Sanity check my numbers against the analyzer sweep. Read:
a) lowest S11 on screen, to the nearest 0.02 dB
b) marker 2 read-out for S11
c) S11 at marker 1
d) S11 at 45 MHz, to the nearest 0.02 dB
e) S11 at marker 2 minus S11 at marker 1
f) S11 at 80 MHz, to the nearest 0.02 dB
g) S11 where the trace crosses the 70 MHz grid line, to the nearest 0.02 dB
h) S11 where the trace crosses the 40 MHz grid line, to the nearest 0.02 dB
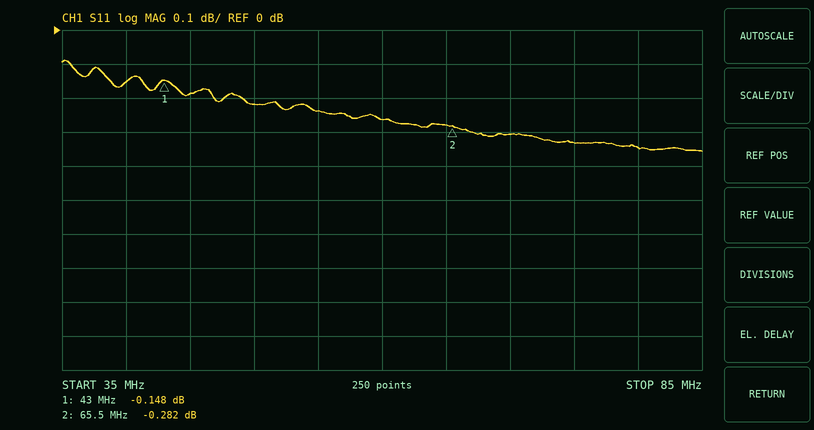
-0.36 dB
-0.282 dB
-0.148 dB
-0.18 dB
-0.134 dB
-0.34 dB
-0.30 dB
-0.16 dB
